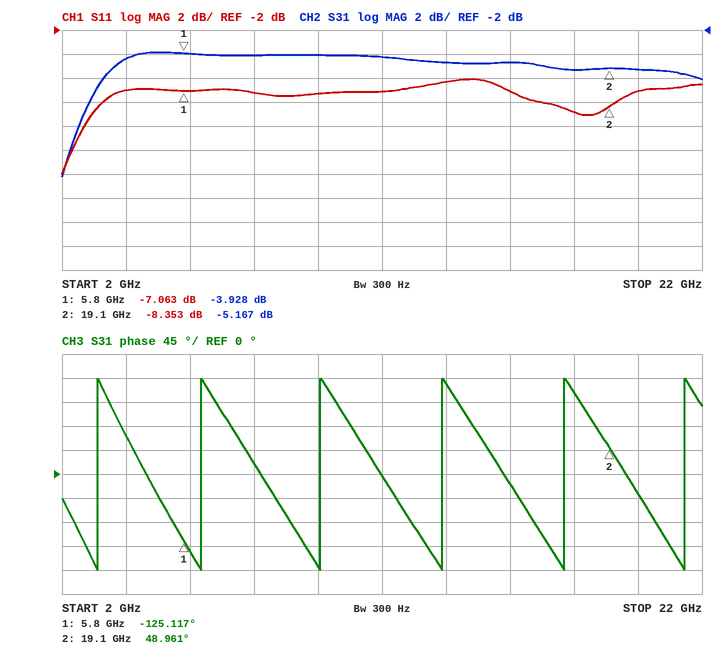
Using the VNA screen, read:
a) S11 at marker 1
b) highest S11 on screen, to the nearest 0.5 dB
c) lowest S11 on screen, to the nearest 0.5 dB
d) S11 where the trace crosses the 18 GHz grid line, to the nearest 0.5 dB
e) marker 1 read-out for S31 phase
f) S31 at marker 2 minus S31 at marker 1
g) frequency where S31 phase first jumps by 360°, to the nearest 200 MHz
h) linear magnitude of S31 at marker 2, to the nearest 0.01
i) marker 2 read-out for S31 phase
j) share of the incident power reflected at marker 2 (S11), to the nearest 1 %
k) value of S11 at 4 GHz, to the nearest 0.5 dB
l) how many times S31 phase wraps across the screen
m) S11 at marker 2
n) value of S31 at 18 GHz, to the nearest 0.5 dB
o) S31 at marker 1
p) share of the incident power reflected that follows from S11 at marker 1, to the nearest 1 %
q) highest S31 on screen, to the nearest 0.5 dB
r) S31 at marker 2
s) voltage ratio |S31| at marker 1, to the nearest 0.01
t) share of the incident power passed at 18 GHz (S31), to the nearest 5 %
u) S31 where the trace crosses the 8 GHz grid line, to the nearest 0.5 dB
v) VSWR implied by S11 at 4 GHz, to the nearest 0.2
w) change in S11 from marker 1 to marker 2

-7.063 dB
-6.0 dB
-14.0 dB
-9.0 dB
-125.117°
-1.239 dB
3.2 GHz
0.55
48.961°
15 %
-7.0 dB
6
-8.353 dB
-5.5 dB
-3.928 dB
20 %
-4.0 dB
-5.167 dB
0.64
30 %
-4.0 dB
2.6
-1.290 dB
